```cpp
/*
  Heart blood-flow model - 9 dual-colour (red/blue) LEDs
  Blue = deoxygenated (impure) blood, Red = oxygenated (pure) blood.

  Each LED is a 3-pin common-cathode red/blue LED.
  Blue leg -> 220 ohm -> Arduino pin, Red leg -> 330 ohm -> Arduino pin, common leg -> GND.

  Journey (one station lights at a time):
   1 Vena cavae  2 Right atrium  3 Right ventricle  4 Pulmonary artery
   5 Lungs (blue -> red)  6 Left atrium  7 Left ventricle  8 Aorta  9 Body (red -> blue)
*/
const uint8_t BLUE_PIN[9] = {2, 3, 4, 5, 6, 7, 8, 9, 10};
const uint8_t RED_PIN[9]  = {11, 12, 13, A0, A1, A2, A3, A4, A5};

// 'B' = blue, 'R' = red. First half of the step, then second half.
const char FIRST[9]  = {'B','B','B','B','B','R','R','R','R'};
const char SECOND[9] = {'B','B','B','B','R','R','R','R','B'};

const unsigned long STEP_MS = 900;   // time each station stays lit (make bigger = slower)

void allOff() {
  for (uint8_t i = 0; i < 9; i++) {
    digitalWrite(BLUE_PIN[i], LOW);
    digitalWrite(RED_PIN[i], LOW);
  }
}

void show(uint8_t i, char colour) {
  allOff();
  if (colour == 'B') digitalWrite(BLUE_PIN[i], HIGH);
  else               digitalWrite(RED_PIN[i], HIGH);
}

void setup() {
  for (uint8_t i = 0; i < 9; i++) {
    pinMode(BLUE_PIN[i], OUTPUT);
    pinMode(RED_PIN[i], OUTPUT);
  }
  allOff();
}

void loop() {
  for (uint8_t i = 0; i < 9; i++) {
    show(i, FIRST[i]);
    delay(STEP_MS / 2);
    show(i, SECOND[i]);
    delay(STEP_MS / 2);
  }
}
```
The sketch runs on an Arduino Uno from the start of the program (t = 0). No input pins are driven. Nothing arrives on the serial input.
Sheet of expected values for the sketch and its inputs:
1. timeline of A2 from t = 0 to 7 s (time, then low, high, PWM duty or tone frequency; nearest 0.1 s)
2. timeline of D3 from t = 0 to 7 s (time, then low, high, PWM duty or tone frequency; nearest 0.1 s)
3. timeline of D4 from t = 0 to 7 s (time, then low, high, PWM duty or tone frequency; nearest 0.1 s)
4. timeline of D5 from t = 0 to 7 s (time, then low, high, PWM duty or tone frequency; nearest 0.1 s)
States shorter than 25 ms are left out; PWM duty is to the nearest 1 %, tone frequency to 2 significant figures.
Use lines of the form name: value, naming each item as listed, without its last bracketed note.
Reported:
timeline of A2 from t = 0 to 7 s: 0 s low; 4.5 s high; 5.4 s low
timeline of D3 from t = 0 to 7 s: 0 s low; 0.9 s high; 1.8 s low
timeline of D4 from t = 0 to 7 s: 0 s low; 1.8 s high; 2.7 s low
timeline of D5 from t = 0 to 7 s: 0 s low; 2.7 s high; 3.6 s low
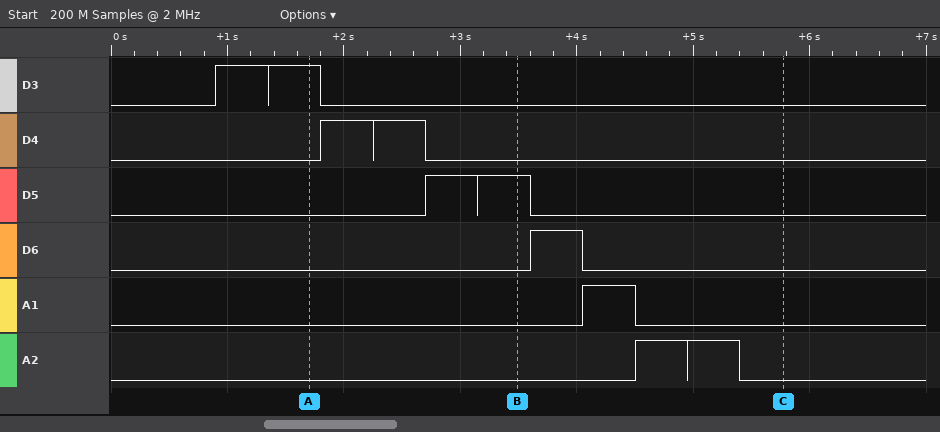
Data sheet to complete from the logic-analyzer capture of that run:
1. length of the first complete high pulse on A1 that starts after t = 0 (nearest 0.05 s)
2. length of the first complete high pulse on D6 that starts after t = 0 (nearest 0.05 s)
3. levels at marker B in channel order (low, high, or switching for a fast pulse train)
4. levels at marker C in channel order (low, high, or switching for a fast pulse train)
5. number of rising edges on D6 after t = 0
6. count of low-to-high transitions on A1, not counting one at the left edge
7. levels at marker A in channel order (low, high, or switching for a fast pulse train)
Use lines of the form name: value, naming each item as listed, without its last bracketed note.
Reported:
length of the first complete high pulse on A1 that starts after t = 0: 0.45 s
length of the first complete high pulse on D6 that starts after t = 0: 0.45 s
levels at marker B in channel order: D3 low, D4 low, D5 high, D6 low, A1 low, A2 low
levels at marker C in channel order: D3 low, D4 low, D5 low, D6 low, A1 low, A2 low
number of rising edges on D6 after t = 0: 1
count of low-to-high transitions on A1, not counting one at the left edge: 1
levels at marker A in channel order: D3 high, D4 low, D5 low, D6 low, A1 low, A2 low
